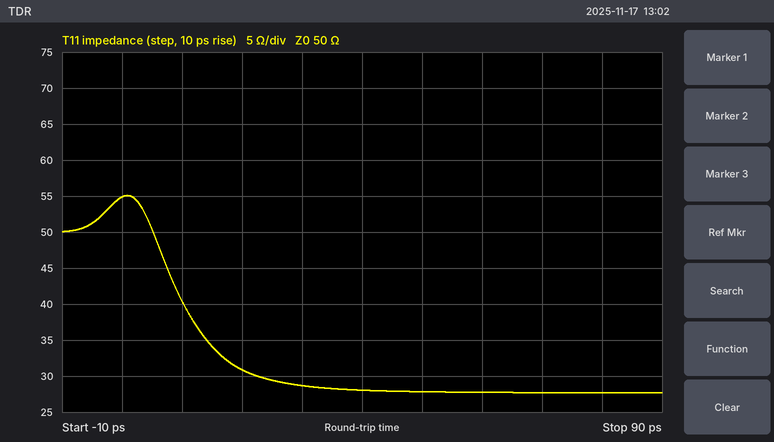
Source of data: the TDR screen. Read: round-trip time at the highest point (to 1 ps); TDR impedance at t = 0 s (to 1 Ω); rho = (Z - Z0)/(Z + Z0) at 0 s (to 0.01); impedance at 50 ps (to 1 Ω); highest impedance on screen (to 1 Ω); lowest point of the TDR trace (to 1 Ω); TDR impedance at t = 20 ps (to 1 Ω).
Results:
1 ps
55 Ω
+0.05
28 Ω
55 Ω
28 Ω
31 Ω
